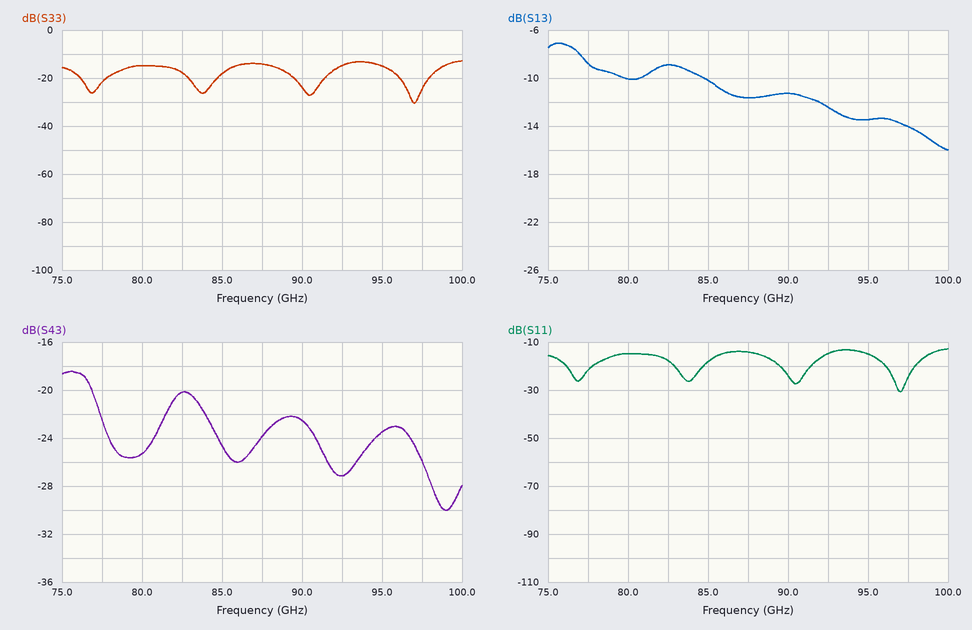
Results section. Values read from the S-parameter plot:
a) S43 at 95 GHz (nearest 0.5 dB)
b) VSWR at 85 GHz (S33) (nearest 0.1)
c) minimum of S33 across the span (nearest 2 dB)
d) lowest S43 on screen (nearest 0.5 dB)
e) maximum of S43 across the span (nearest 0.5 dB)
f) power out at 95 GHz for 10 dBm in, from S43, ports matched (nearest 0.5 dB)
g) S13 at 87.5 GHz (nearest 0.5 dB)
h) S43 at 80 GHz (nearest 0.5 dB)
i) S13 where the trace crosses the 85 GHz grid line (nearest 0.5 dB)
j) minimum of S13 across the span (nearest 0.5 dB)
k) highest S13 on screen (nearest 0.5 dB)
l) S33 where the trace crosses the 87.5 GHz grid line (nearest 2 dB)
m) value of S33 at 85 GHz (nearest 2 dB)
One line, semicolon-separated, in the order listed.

-23.5 dB; 1.3; -30 dB; -30.0 dB; -18.5 dB; -13.5 dBm; -11.5 dB; -25.5 dB; -10.0 dB; -16.0 dB; -7.0 dB; -14 dB; -18 dB
